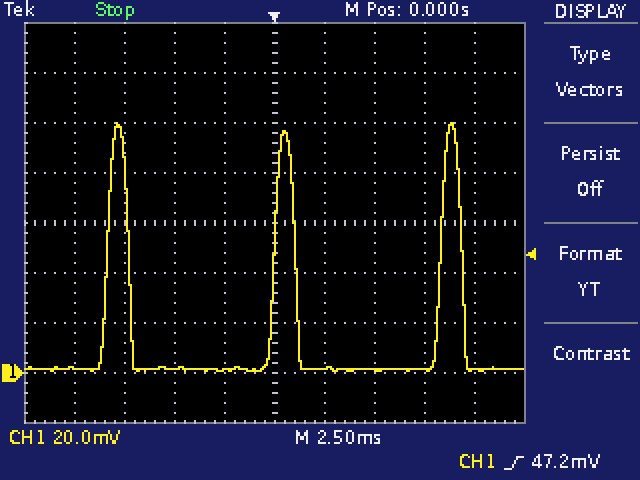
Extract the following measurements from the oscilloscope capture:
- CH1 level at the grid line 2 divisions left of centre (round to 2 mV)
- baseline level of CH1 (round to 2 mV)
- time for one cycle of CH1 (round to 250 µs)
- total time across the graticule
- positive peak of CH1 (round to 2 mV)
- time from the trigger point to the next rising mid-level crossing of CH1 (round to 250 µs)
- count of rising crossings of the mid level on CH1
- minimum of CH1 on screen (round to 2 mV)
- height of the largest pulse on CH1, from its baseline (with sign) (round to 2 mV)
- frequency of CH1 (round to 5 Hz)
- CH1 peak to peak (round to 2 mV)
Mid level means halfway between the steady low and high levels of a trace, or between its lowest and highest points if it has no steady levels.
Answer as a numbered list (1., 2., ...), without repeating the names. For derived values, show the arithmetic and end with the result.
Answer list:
1. 2 mV
2. 2 mV
3. 8.25 ms
4. 25 ms
5. 100 mV
6. 8.25 ms
7. 3
8. 0 mV
9. 100 mV − (2 mV) = +98 mV
10. 1 / 8.25 ms ≈ 121 Hz, so 120 Hz to the nearest 5 Hz
11. 100 mV − (0 mV) = 100 mV
